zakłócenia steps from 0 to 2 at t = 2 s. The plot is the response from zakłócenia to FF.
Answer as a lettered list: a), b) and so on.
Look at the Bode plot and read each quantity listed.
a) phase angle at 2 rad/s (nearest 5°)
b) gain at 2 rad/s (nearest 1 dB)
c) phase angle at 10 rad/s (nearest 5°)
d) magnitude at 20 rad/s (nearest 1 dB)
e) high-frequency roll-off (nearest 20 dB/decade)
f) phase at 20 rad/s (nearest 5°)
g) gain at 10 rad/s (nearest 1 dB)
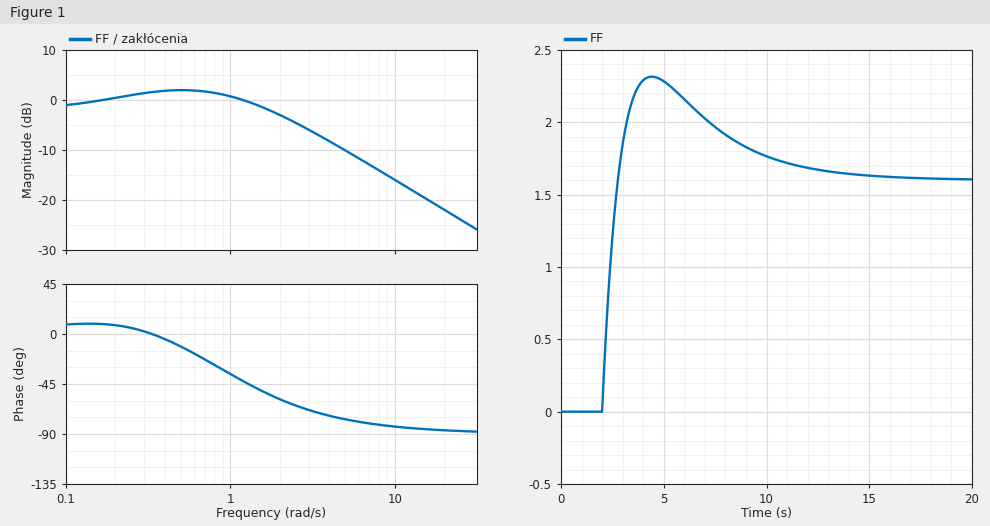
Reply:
a) -60°
b) -3 dB
c) -85°
d) -22 dB
e) -20 dB/decade
f) -85°
g) -16 dB
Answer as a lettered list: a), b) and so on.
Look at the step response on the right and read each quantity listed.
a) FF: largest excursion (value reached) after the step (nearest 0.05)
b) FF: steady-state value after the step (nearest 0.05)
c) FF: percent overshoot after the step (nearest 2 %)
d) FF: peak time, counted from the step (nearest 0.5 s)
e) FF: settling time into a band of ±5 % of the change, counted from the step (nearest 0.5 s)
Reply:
a) 2.30
b) 1.60
c) 44 %
d) 2.5 s
e) 10.0 s
